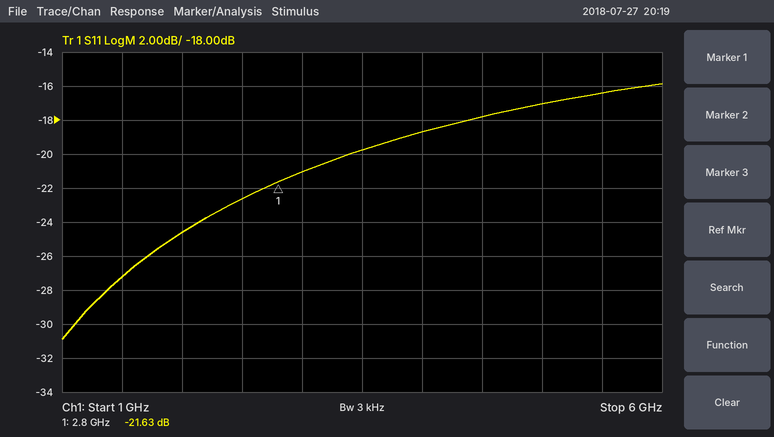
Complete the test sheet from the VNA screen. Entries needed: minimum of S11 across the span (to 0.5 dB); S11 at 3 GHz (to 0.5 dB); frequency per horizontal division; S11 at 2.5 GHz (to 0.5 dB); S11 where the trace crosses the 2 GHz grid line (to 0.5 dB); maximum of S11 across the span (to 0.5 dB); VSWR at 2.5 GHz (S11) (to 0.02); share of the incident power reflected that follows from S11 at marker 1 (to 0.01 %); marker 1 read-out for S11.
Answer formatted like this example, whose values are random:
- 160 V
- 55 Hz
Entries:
- -31.0 dB
- -21.0 dB
- 500 MHz
- -22.5 dB
- -24.5 dB
- -16.0 dB
- 1.16
- 0.69 %
- -21.63 dB
